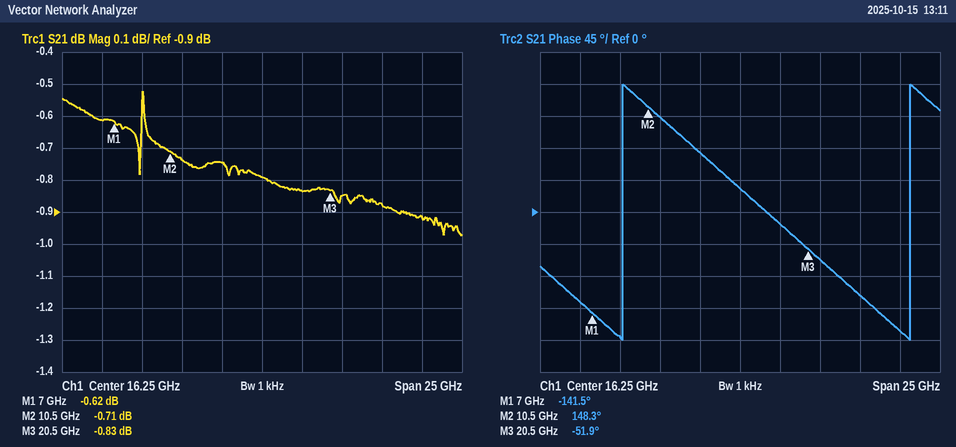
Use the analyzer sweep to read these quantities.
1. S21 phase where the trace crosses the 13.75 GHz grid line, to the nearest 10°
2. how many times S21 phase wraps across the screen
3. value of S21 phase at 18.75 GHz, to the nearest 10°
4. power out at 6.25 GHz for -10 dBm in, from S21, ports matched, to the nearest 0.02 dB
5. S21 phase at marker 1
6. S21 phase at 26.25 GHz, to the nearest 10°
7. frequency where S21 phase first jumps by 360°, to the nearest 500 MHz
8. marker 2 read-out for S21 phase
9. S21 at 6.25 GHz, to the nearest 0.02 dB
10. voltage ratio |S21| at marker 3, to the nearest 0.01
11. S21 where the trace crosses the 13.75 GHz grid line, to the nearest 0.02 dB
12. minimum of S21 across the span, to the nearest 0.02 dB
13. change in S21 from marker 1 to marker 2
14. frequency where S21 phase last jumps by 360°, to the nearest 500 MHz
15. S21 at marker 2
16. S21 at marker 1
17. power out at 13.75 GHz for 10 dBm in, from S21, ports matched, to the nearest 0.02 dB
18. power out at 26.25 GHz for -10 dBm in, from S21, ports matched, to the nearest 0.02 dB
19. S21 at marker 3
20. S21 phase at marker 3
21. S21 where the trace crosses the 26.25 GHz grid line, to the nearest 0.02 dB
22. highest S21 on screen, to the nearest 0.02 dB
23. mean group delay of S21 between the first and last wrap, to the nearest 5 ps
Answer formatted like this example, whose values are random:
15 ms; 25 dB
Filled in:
80°; 2; -20°; -10.62 dBm; -141.5°; -170°; 9.0 GHz; 148.3°; -0.62 dB; 0.91; -0.74 dB; -0.98 dB; -0.09 dB; 27.0 GHz; -0.71 dB; -0.62 dB; 9.26 dBm; -10.92 dBm; -0.83 dB; -51.9°; -0.92 dB; -0.52 dB; 55 ps
